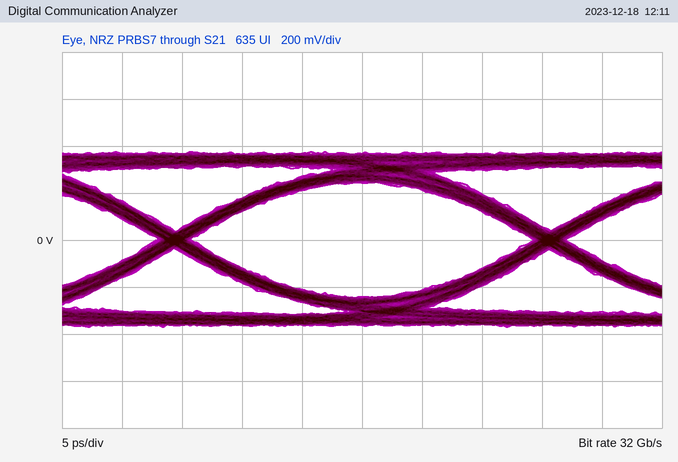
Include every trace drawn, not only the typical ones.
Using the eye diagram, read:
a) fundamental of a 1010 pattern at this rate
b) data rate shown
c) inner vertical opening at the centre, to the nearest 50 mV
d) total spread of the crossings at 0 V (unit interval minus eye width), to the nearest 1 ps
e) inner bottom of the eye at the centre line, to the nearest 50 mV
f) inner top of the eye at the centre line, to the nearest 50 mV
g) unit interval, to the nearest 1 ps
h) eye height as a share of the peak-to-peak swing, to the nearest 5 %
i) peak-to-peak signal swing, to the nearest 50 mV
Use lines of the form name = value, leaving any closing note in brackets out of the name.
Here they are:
fundamental of a 1010 pattern at this rate = 16 GHz
data rate shown = 32 Gb/s
inner vertical opening at the centre, to the nearest 50 mV = 500 mV
total spread of the crossings at 0 V (unit interval minus eye width), to the nearest 1 ps = 3 ps
inner bottom of the eye at the centre line, to the nearest 50 mV = -250 mV
inner top of the eye at the centre line, to the nearest 50 mV = 250 mV
unit interval, to the nearest 1 ps = 31 ps
eye height as a share of the peak-to-peak swing, to the nearest 5 % = 65 %
peak-to-peak signal swing, to the nearest 50 mV = 750 mV
